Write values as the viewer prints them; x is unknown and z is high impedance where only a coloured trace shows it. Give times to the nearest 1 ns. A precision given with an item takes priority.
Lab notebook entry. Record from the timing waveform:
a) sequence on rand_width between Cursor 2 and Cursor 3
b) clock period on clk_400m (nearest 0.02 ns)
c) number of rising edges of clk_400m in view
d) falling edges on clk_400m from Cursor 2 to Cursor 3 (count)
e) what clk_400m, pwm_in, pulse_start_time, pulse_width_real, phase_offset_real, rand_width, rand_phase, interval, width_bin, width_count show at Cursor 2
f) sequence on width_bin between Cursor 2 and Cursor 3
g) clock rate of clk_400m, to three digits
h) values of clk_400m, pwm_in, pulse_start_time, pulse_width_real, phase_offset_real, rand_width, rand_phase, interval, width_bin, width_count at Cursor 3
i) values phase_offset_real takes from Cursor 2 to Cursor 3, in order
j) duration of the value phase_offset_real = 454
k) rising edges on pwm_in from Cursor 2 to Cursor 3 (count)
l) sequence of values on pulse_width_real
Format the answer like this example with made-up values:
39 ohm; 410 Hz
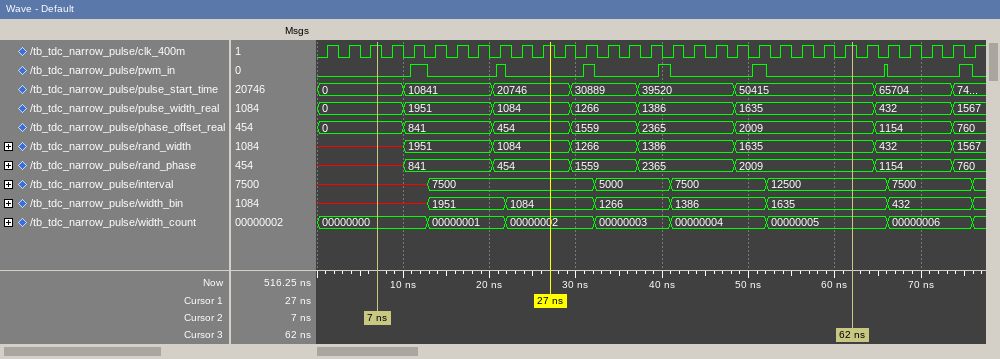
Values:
x, 1951, 1084, 1266, 1386, 1635; 2.5 ns; 31; 22; clk_400m=1, pwm_in=0, pulse_start_time=0, pulse_width_real=0, phase_offset_real=0, rand_width=x, rand_phase=x, interval=x, width_bin=x, width_count=00000000; x, 1951, 1084, 1266, 1386, 1635; 400 MHz; clk_400m=1, pwm_in=0, pulse_start_time=50415, pulse_width_real=1635, phase_offset_real=2009, rand_width=1635, rand_phase=2009, interval=12500, width_bin=1635, width_count=00000005; 0, 841, 454, 1559, 2365, 2009; 9 ns; 5; 0, 1951, 1084, 1266, 1386, 1635, 432, 1567
